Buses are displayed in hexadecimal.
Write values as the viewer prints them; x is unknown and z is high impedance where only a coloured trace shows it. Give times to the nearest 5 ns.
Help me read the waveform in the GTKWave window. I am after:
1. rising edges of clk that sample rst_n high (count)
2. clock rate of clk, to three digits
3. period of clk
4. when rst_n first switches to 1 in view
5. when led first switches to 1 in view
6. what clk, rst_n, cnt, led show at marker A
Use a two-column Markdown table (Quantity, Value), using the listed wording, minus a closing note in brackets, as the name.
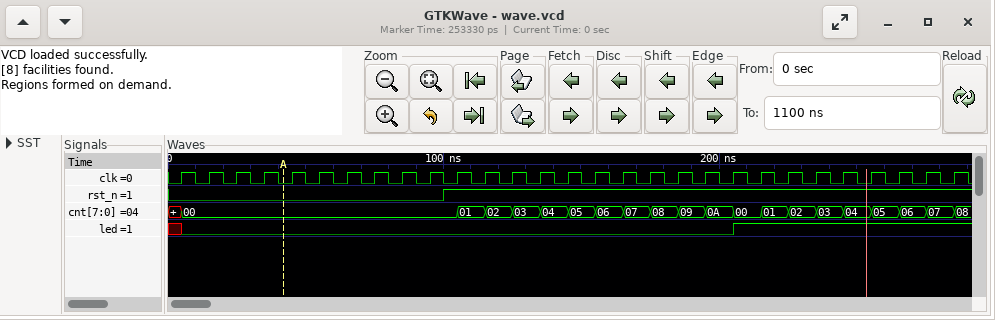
| Quantity | Value |
|---|---|
| rising edges of clk that sample rst_n high | 19 |
| clock rate of clk, to three digits | 100 MHz |
| period of clk | 10 ns |
| when rst_n first switches to 1 in view | 100 ns |
| when led first switches to 1 in view | 205 ns |
| what clk, rst_n, cnt, led show at marker A | clk=0, rst_n=0, cnt=00, led=0 |
